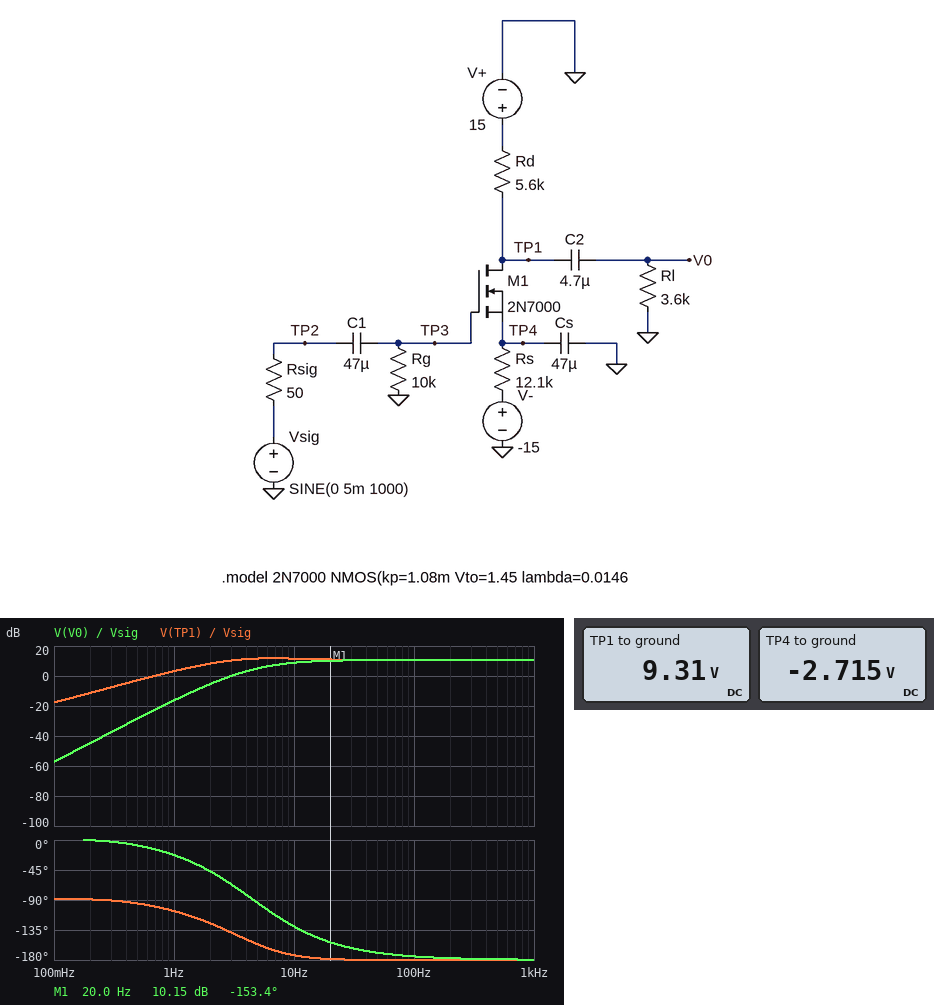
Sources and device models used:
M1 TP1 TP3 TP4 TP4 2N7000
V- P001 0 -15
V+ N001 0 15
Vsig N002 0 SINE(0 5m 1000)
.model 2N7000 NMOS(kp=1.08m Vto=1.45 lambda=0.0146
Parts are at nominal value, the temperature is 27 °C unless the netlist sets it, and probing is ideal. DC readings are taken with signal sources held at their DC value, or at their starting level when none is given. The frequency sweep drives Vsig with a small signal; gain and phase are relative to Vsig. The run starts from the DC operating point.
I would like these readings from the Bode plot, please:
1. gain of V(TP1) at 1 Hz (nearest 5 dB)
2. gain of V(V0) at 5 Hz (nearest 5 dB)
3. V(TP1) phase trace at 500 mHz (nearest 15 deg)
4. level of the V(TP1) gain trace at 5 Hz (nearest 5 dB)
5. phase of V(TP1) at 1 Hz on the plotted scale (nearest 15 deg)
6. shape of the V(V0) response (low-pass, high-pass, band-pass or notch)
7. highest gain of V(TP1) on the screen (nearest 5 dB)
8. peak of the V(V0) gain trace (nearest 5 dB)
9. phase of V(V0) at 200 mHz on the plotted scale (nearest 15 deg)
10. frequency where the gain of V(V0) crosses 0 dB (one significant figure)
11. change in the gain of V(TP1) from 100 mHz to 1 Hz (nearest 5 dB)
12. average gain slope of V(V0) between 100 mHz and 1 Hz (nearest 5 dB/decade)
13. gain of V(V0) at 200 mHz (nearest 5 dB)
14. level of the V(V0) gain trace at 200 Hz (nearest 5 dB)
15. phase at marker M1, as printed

5 dB
5 dB
-90 deg
10 dB
-105 deg
high-pass
10 dB
10 dB
0 deg
3 Hz
20 dB
40 dB/decade
-45 dB
10 dB
-153.4 deg
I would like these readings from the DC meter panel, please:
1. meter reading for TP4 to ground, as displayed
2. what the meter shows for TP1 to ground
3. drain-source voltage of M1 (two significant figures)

-2.715 V
9.31 V
12 V
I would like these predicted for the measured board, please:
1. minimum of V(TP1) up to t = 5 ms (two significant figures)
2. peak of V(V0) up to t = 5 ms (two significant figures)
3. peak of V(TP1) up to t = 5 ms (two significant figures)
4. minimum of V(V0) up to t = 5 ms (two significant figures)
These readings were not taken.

9.3 V
17 mV
9.3 V
-17 mV
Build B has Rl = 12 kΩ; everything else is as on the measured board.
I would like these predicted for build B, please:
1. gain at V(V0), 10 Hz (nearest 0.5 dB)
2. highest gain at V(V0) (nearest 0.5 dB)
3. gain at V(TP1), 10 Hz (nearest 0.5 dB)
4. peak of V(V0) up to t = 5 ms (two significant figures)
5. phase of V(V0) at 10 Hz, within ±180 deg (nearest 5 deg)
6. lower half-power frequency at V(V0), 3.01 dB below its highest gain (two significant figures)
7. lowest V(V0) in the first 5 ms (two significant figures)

14.0 dB
15.5 dB
14.5 dB
29 mV
-140 deg
6.1 Hz
-29 mV
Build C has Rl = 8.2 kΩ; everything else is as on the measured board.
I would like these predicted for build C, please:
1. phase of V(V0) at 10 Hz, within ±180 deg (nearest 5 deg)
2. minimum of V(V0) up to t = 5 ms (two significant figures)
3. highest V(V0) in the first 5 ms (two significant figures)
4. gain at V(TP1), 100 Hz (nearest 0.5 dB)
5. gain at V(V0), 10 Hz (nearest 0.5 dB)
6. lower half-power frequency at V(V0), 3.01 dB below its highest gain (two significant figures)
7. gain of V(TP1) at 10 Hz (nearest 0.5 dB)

-135 deg
-25 mV
26 mV
14.0 dB
12.5 dB
6.5 Hz
13.5 dB
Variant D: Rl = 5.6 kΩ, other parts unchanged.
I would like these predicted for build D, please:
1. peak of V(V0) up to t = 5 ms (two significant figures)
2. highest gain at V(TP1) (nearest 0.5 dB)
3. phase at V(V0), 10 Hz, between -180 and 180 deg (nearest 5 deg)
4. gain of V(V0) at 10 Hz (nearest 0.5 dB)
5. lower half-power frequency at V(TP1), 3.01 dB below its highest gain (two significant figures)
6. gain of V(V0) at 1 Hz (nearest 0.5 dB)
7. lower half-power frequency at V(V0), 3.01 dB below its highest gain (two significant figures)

22 mV
12.5 dB
-135 deg
11.0 dB
2.7 Hz
-12.5 dB
6.9 Hz
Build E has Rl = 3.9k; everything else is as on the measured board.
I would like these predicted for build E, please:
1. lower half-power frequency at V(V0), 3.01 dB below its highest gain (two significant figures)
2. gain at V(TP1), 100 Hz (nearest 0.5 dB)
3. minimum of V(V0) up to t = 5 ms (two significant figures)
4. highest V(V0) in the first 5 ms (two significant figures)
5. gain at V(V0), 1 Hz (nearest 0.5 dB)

7.4 Hz
11.0 dB
-18 mV
18 mV
-15.5 dB
